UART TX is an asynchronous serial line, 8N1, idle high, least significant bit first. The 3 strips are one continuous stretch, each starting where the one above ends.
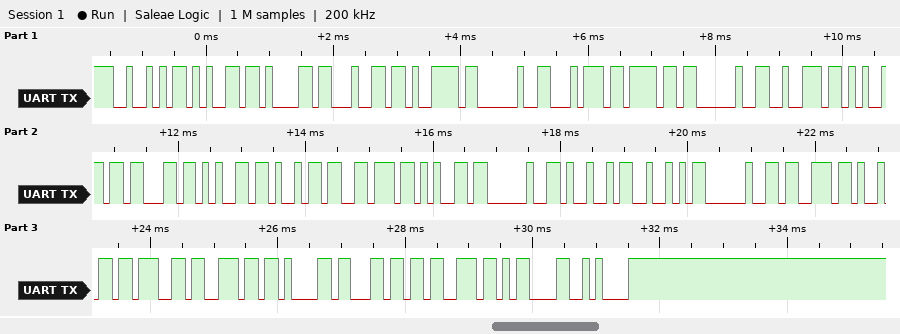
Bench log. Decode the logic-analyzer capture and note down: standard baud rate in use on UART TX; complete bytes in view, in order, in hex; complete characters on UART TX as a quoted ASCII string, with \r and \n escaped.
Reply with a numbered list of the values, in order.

1. 9600 baud
2. 52 65 61 64 79 20 74 6F 20 72 65 63 65 69 76 65 20 49 52 20 73 69 67 6E 61 6C 73 0D 0A
3. "Ready to receive IR signals\r\n"
